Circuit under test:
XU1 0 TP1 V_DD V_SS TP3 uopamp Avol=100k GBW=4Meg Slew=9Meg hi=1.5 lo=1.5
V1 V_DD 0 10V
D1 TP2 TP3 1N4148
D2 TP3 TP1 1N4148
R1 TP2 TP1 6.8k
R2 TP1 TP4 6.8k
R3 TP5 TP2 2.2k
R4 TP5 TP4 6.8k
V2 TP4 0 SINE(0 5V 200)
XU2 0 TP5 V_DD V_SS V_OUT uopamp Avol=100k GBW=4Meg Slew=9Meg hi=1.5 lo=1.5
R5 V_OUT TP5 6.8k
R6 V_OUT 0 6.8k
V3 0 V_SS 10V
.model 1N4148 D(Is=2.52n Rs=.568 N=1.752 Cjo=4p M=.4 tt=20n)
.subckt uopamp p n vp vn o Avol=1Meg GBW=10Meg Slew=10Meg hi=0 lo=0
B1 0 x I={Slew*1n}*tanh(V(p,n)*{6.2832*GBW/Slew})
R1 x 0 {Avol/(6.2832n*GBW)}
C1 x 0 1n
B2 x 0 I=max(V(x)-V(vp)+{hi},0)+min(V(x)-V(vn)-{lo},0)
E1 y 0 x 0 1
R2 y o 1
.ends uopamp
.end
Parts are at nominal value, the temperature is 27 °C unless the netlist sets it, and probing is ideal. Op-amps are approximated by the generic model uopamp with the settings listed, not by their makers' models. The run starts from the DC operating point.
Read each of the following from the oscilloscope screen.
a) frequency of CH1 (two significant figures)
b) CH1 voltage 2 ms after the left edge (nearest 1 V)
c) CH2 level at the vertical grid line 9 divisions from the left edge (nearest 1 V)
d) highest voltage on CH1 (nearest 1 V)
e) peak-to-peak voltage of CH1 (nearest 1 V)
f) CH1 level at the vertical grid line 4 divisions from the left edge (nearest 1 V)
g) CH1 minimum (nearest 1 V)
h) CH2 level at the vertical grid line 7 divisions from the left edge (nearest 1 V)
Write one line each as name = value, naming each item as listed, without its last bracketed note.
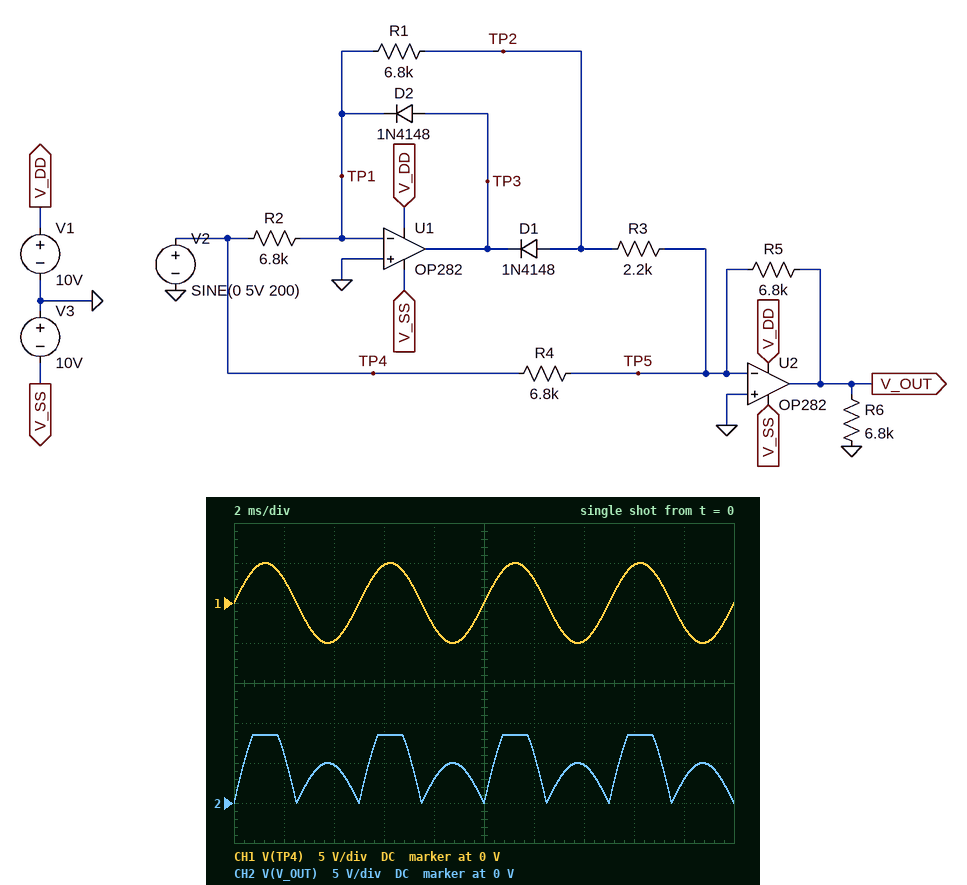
frequency of CH1 = 200 Hz
CH1 voltage 2 ms after the left edge = 3 V
CH2 level at the vertical grid line 9 divisions from the left edge = 3 V
highest voltage on CH1 = 5 V
peak-to-peak voltage of CH1 = 10 V
CH1 level at the vertical grid line 4 divisions from the left edge = -3 V
CH1 minimum = -5 V
CH2 level at the vertical grid line 7 divisions from the left edge = 5 V
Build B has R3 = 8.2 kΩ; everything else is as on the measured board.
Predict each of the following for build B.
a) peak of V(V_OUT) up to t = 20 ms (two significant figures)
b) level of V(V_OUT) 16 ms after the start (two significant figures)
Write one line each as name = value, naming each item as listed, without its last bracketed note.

peak of V(V_OUT) up to t = 20 ms = 5.0 V
level of V(V_OUT) 16 ms after the start = -810 mV
